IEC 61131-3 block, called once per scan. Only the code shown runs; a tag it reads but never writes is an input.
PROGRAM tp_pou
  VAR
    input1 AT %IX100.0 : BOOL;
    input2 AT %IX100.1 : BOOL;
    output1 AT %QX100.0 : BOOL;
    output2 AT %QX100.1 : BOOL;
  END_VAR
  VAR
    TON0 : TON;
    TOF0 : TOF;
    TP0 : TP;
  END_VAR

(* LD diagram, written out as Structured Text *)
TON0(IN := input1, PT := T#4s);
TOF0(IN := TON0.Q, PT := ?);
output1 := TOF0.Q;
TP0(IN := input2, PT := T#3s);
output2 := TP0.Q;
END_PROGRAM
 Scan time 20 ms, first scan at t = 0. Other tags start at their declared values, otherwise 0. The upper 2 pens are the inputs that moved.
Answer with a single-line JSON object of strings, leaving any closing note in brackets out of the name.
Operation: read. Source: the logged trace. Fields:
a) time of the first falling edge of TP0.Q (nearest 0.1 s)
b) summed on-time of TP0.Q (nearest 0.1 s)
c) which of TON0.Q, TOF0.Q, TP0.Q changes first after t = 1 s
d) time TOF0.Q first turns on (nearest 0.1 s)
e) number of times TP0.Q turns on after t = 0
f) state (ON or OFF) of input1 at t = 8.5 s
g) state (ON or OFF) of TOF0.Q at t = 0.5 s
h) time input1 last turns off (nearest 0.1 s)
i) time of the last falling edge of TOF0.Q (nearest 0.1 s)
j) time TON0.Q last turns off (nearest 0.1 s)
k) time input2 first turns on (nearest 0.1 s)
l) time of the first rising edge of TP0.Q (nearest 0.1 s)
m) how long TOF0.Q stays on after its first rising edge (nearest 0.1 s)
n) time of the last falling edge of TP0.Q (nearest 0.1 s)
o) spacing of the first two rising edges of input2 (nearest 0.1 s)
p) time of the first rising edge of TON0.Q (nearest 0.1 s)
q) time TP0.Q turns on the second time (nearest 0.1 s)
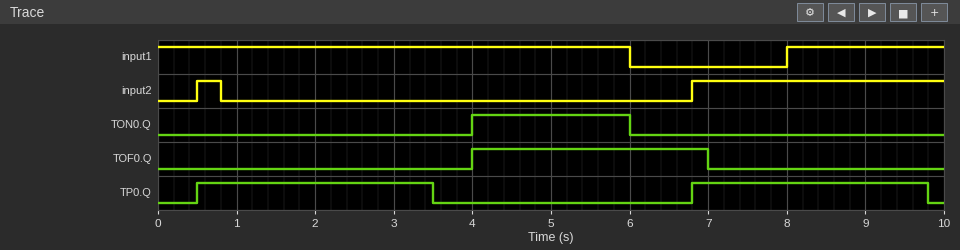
{"time of the first falling edge of TP0.Q": "3.5 s", "summed on-time of TP0.Q": "6.0 s", "which of TON0.Q, TOF0.Q, TP0.Q changes first after t = 1 s": "TP0.Q", "time TOF0.Q first turns on": "4.0 s", "number of times TP0.Q turns on after t = 0": "2", "state (ON or OFF) of input1 at t = 8.5 s": "ON", "state (ON or OFF) of TOF0.Q at t = 0.5 s": "OFF", "time input1 last turns off": "6.0 s", "time of the last falling edge of TOF0.Q": "7.0 s", "time TON0.Q last turns off": "6.0 s", "time input2 first turns on": "0.5 s", "time of the first rising edge of TP0.Q": "0.5 s", "how long TOF0.Q stays on after its first rising edge": "3.0 s", "time of the last falling edge of TP0.Q": "9.8 s", "spacing of the first two rising edges of input2": "6.3 s", "time of the first rising edge of TON0.Q": "4.0 s", "time TP0.Q turns on the second time": "6.8 s"}
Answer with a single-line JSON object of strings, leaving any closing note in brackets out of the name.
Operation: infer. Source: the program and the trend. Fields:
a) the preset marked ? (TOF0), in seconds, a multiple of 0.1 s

{"the preset marked ? (TOF0), in seconds, a multiple of 0.1 s": "1.0 s"}
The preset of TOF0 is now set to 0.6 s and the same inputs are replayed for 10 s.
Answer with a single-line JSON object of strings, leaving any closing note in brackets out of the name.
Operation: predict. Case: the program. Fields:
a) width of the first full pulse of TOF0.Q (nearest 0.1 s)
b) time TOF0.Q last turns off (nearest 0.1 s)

{"width of the first full pulse of TOF0.Q": "2.6 s", "time TOF0.Q last turns off": "6.6 s"}
